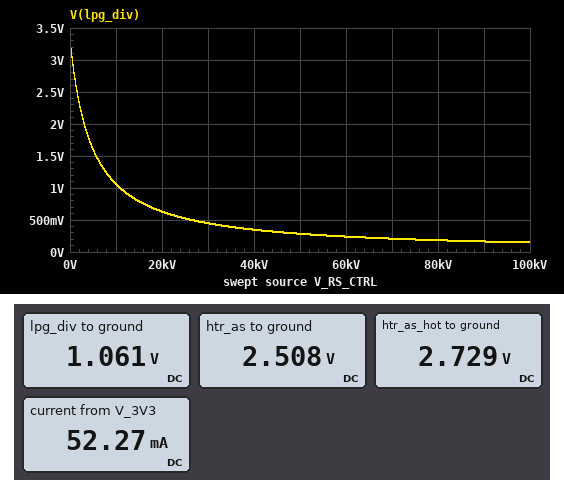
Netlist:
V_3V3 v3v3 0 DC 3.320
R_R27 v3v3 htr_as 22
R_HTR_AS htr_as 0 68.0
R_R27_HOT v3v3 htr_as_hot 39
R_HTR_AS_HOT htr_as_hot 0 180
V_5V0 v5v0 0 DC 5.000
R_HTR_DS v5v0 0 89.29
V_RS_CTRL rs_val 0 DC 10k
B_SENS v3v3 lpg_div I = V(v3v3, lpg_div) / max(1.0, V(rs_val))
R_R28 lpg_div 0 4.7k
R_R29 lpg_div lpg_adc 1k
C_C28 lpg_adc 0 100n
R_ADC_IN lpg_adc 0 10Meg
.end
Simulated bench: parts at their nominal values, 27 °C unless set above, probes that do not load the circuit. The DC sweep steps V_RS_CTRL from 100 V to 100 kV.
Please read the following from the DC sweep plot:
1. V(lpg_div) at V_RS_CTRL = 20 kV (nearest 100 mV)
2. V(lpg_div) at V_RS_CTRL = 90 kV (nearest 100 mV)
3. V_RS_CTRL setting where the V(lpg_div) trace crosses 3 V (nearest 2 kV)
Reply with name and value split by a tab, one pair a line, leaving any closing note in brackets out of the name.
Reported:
V(lpg_div) at V_RS_CTRL = 20 kV	600 mV
V(lpg_div) at V_RS_CTRL = 90 kV	200 mV
V_RS_CTRL setting where the V(lpg_div) trace crosses 3 V	0 V
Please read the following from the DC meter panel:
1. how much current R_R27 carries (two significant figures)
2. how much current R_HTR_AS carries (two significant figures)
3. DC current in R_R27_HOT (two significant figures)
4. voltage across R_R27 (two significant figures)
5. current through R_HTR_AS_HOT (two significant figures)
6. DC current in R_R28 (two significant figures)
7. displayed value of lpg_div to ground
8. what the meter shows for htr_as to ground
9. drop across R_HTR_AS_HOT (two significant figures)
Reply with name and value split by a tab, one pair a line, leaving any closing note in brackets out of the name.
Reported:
how much current R_R27 carries	37 mA
how much current R_HTR_AS carries	37 mA
DC current in R_R27_HOT	15 mA
voltage across R_R27	810 mV
current through R_HTR_AS_HOT	15 mA
DC current in R_R28	230 µA
displayed value of lpg_div to ground	1.061 V
what the meter shows for htr_as to ground	2.508 V
drop across R_HTR_AS_HOT	2.7 V
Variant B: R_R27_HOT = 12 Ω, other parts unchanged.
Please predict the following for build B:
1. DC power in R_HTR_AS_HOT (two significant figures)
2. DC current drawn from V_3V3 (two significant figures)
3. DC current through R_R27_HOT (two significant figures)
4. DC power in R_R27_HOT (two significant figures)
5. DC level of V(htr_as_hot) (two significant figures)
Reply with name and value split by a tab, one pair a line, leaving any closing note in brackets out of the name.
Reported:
DC power in R_HTR_AS_HOT	54 mW
DC current drawn from V_3V3	54 mA
DC current through R_R27_HOT	17 mA
DC power in R_R27_HOT	3.6 mW
DC level of V(htr_as_hot)	3.1 V
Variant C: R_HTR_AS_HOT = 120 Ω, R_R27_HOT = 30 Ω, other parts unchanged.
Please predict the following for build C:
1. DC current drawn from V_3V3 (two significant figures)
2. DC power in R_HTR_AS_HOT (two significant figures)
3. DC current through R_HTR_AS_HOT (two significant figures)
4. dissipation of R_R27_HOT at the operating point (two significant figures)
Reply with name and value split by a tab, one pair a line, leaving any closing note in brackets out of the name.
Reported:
DC current drawn from V_3V3	59 mA
DC power in R_HTR_AS_HOT	59 mW
DC current through R_HTR_AS_HOT	22 mA
dissipation of R_R27_HOT at the operating point	15 mW
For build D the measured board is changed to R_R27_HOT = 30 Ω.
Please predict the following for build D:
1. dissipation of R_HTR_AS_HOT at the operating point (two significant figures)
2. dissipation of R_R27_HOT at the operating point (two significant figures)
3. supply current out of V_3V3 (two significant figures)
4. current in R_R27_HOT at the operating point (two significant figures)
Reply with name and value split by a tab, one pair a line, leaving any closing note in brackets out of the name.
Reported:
dissipation of R_HTR_AS_HOT at the operating point	45 mW
dissipation of R_R27_HOT at the operating point	7.5 mW
supply current out of V_3V3	53 mA
current in R_R27_HOT at the operating point	16 mA
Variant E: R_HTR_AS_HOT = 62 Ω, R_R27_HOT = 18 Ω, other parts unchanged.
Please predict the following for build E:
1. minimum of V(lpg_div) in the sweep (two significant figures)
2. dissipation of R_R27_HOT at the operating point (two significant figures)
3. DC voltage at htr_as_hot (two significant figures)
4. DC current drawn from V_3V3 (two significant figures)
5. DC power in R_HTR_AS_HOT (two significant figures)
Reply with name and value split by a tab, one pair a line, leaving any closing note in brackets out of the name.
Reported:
minimum of V(lpg_div) in the sweep	150 mV
dissipation of R_R27_HOT at the operating point	31 mW
DC voltage at htr_as_hot	2.6 V
DC current drawn from V_3V3	79 mA
DC power in R_HTR_AS_HOT	110 mW
